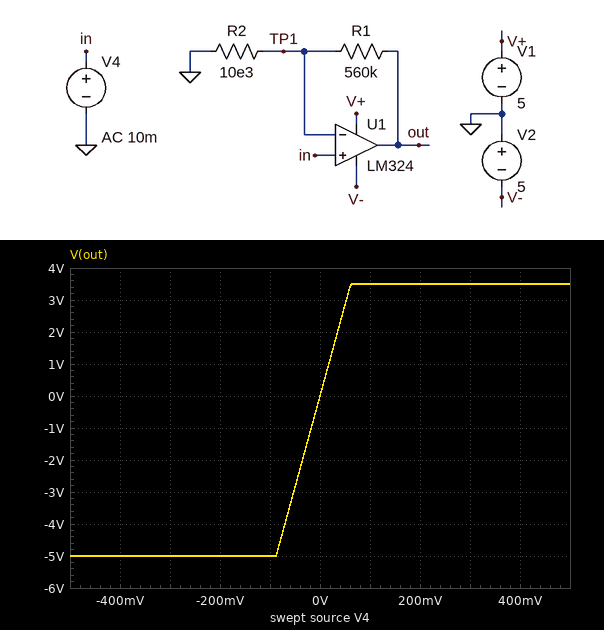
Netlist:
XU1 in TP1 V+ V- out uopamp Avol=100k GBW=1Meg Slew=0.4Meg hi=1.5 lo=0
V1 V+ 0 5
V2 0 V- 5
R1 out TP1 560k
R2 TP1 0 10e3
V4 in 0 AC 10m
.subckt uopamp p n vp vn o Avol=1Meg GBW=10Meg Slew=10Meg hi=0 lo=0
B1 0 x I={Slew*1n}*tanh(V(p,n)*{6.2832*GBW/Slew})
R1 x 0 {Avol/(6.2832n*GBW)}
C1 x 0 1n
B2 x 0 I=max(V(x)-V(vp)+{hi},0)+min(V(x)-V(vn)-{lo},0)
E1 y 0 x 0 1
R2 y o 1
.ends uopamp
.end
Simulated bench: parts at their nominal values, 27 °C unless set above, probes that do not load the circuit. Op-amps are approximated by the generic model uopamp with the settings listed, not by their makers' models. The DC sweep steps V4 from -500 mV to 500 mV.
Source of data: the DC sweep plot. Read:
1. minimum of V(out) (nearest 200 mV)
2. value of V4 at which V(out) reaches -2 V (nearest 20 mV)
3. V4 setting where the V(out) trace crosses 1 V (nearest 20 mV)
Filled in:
-5.0 V
-40 mV
20 mV
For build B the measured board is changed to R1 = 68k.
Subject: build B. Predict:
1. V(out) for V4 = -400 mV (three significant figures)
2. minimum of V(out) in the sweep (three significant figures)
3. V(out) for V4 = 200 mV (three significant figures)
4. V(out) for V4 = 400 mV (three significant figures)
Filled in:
-3.12 V
-3.90 V
1.56 V
3.12 V
